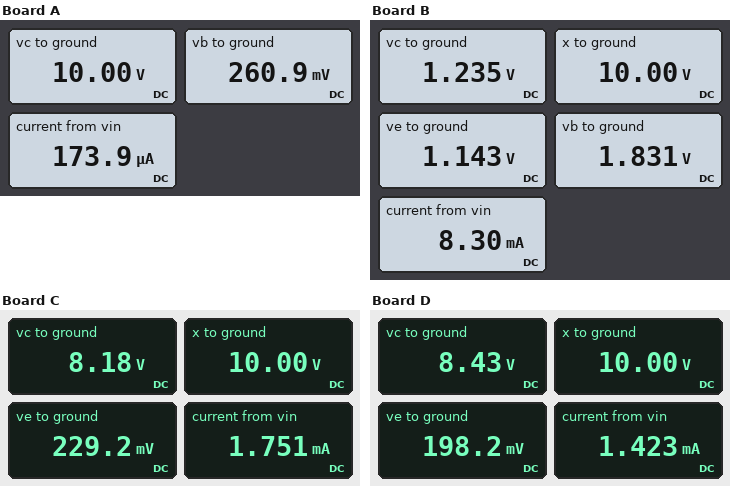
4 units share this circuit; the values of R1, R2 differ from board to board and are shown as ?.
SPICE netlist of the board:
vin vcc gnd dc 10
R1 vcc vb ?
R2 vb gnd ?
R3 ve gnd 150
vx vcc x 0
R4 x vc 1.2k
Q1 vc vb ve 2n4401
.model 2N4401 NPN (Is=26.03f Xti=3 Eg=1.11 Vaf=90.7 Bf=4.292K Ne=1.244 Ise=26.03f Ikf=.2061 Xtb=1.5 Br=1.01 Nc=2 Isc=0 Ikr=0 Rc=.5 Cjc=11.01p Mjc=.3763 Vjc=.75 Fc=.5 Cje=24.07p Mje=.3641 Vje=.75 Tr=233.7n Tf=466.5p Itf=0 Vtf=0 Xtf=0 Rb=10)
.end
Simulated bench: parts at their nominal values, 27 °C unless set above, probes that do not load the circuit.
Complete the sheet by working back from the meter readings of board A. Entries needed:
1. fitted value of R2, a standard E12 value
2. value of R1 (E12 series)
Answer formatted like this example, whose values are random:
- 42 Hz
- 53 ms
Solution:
- 1.5 kΩ
- 56 kΩ
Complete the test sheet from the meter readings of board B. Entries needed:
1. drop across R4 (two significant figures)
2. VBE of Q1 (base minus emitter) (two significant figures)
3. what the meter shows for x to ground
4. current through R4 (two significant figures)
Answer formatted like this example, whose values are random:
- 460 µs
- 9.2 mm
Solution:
- 8.8 V
- 690 mV
- 10.00 V
- 7.3 mA
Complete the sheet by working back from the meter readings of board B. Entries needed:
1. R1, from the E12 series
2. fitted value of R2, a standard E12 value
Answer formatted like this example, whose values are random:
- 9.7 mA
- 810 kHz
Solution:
- 8.2 kΩ
- 2.7 kΩ
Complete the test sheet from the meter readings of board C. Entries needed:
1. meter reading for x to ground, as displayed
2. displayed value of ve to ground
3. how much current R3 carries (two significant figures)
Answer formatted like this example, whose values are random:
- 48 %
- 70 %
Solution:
- 10.00 V
- 229.2 mV
- 1.5 mA
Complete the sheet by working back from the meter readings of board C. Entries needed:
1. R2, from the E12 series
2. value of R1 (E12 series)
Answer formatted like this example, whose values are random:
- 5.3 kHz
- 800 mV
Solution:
- 3.9 kΩ
- 39 kΩ
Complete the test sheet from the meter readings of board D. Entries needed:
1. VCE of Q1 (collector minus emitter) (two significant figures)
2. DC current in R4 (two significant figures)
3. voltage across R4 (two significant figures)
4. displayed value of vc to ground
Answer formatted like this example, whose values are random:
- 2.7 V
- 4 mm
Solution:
- 8.2 V
- 1.3 mA
- 1.6 V
- 8.43 V
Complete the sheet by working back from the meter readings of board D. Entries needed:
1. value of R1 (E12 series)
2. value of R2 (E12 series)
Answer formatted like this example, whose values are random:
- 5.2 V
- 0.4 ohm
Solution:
- 82 kΩ
- 8.2 kΩ
